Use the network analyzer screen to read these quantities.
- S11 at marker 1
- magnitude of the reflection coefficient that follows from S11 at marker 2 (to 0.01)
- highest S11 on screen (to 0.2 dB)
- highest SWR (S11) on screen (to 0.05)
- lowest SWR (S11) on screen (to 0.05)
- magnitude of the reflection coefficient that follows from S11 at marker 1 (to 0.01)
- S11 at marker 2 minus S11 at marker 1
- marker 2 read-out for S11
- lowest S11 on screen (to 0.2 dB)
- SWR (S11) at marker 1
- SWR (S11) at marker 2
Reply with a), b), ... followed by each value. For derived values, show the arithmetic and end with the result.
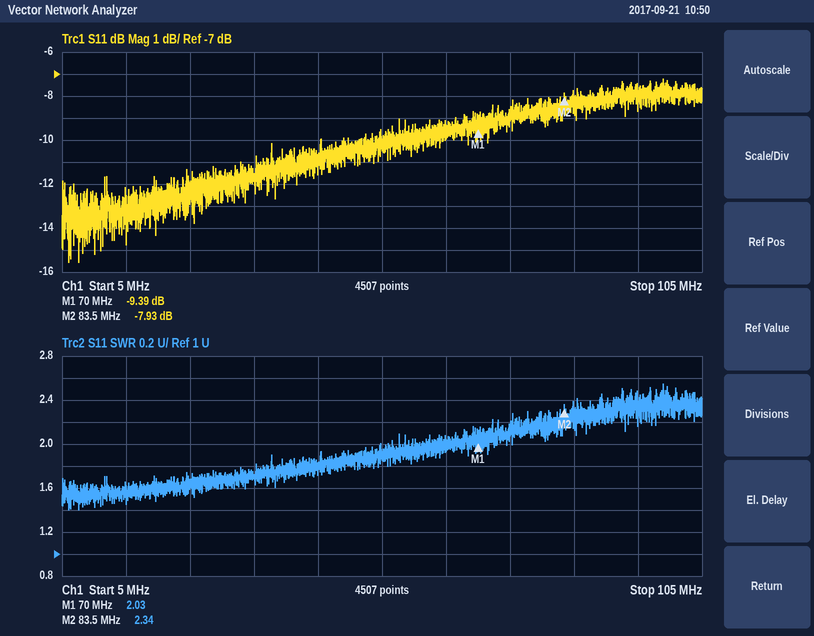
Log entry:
a) -9.39 dB
b) 10^(-7.93/20) ≈ 0.40
c) -7.2 dB
d) 2.55
e) 1.40
f) 10^(-9.39/20) ≈ 0.34
g) -7.93 − (-9.39) = 1.46 dB
h) -7.93 dB
i) -15.6 dB
j) 2.03
k) 2.34
